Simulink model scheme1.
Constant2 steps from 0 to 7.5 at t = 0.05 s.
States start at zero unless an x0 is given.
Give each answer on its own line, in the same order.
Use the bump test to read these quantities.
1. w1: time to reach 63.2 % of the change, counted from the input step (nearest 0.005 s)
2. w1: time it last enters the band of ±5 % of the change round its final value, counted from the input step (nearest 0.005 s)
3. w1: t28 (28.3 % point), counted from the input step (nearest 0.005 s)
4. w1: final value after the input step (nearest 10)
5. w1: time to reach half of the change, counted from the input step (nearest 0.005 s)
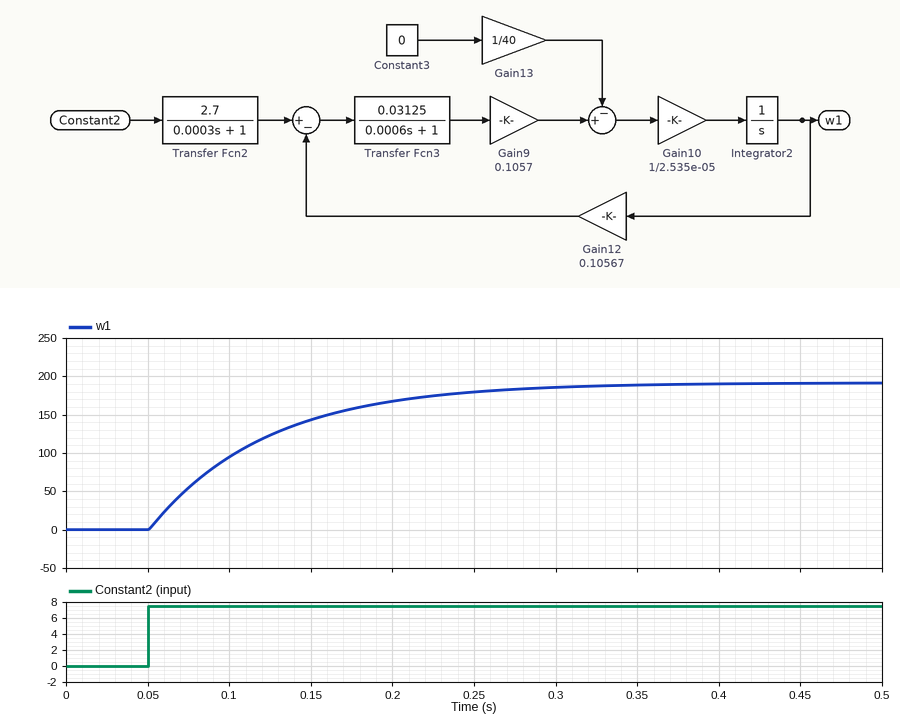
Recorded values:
0.075 s
0.215 s
0.025 s
190
0.050 s
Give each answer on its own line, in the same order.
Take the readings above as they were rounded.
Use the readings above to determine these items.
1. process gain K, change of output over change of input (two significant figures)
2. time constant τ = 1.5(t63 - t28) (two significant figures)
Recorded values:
25
0.075 s
